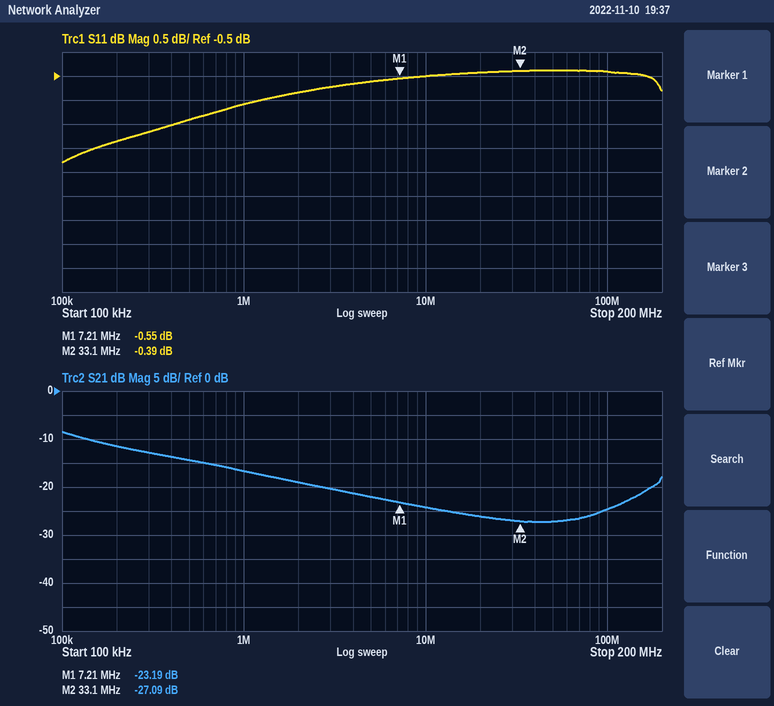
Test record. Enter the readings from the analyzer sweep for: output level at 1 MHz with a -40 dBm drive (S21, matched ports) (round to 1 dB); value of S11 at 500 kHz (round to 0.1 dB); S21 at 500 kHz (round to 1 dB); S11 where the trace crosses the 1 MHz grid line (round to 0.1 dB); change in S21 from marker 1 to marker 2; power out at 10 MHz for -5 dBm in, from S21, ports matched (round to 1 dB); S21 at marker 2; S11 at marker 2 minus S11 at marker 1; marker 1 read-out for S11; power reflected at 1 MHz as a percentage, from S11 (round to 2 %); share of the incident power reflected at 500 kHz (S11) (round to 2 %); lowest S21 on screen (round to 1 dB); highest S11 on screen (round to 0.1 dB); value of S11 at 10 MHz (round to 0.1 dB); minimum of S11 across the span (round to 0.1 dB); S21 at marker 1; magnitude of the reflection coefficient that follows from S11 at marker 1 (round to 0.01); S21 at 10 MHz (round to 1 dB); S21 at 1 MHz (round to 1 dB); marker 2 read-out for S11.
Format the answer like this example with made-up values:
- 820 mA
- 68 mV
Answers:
- -57 dBm
- -1.4 dB
- -14 dB
- -1.1 dB
- -3.90 dB
- -29 dBm
- -27.09 dB
- 0.16 dB
- -0.55 dB
- 78 %
- 72 %
- -27 dB
- -0.4 dB
- -0.5 dB
- -2.3 dB
- -23.19 dB
- 0.94
- -24 dB
- -17 dB
- -0.39 dB
